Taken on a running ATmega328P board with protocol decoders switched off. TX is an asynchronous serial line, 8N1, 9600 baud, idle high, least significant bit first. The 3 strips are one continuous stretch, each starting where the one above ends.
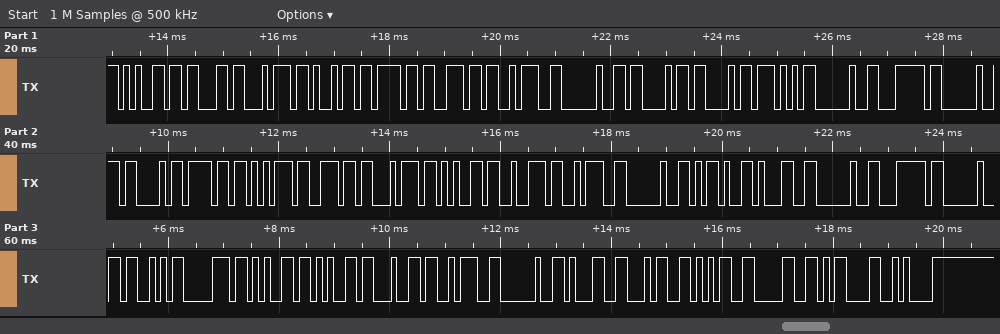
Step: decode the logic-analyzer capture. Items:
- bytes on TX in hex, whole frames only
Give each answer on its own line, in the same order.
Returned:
65 63 74 69 6F 6E 3A 20 43 43 57 20 7C 20 43 6F 75 6E 74 65 72 3A 20 2D 31 20 7C 20 53 70 65 65 64 3A 20 31 34 35 30 0D 0A
